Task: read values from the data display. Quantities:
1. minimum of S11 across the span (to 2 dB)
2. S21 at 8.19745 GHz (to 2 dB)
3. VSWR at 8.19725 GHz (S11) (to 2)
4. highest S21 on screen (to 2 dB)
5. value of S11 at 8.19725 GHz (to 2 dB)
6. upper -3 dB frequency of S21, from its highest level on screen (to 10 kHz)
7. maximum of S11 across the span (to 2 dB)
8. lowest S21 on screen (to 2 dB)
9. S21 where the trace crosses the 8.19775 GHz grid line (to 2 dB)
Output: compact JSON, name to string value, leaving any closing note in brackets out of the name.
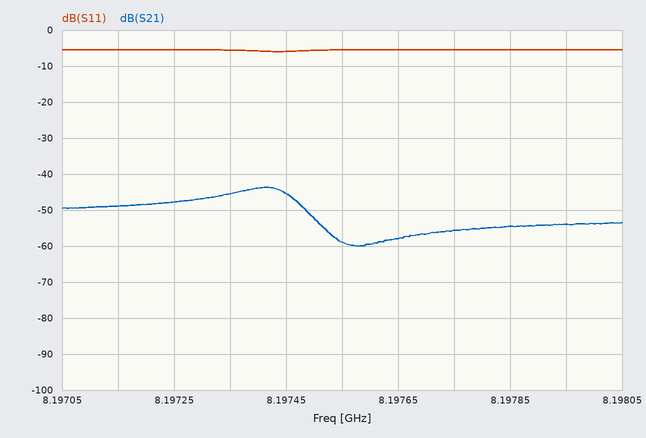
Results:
{"minimum of S11 across the span": "-6 dB", "S21 at 8.19745 GHz": "-46 dB", "VSWR at 8.19725 GHz (S11)": "4", "highest S21 on screen": "-44 dB", "value of S11 at 8.19725 GHz": "-6 dB", "upper -3 dB frequency of S21, from its highest level on screen": "8.19746 GHz", "maximum of S11 across the span": "-6 dB", "lowest S21 on screen": "-60 dB", "S21 where the trace crosses the 8.19775 GHz grid line": "-56 dB"}
